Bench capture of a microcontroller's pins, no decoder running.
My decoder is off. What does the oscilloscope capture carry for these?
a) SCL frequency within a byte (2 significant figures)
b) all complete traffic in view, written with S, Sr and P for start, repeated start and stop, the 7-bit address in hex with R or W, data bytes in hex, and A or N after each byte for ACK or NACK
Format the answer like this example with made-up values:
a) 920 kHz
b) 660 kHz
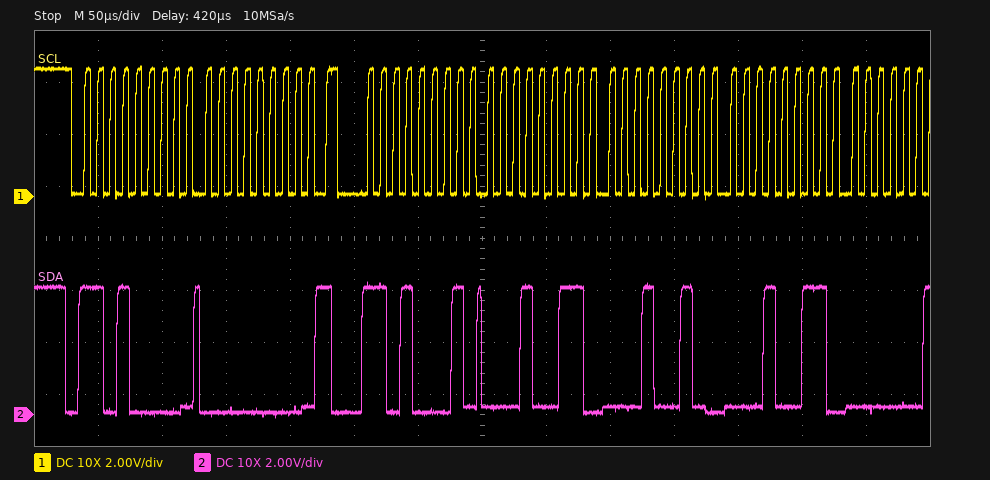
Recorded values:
a) 100 kHz
b) S 68W A 00 A Sr 68R A 13 A 12 A 13 A
